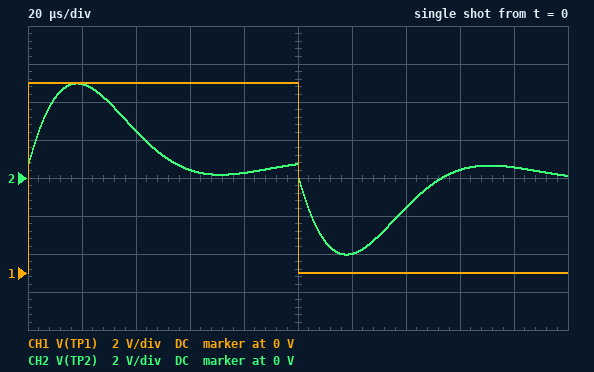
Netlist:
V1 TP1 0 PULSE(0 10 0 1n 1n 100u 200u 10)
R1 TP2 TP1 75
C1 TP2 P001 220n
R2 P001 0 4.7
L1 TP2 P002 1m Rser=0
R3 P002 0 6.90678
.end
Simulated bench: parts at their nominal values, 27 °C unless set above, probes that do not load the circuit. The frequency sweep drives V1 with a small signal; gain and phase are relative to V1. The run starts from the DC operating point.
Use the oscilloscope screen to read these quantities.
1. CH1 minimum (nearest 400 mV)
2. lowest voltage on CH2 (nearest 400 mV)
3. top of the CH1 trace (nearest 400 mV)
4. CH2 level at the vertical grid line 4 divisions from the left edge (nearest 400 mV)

0 V
-4.0 V
10.0 V
400 mV
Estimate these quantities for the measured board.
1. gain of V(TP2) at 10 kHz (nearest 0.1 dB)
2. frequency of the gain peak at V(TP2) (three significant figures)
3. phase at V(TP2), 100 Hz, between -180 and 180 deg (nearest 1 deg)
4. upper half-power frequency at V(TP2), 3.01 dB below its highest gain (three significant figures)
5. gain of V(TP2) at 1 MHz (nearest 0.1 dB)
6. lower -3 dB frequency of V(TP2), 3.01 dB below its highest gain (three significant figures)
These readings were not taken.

-1.6 dB
10.9 kHz
5 deg
17.6 kHz
-24.5 dB
6.68 kHz
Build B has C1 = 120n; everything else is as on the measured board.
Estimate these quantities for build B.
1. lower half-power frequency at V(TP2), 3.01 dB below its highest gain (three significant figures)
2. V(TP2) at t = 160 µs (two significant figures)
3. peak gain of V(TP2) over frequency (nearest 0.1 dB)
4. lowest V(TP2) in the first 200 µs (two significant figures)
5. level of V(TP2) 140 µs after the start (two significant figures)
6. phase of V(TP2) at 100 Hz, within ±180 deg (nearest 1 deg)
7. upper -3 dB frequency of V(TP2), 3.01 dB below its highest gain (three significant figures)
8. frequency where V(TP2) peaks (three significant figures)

8.11 kHz
380 mV
-0.9 dB
-5.0 V
-360 mV
5 deg
26.6 kHz
14.7 kHz
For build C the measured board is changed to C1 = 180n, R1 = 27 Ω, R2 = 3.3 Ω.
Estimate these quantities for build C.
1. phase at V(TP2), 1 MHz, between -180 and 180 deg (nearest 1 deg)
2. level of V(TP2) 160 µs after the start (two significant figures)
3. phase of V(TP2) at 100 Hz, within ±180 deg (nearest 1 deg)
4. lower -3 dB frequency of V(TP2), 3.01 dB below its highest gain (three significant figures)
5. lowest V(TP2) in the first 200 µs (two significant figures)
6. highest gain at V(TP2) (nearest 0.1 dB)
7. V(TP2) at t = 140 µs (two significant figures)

-13 deg
-1.1 V
4 deg
4.29 kHz
-5.7 V
-0.4 dB
-2.5 V
